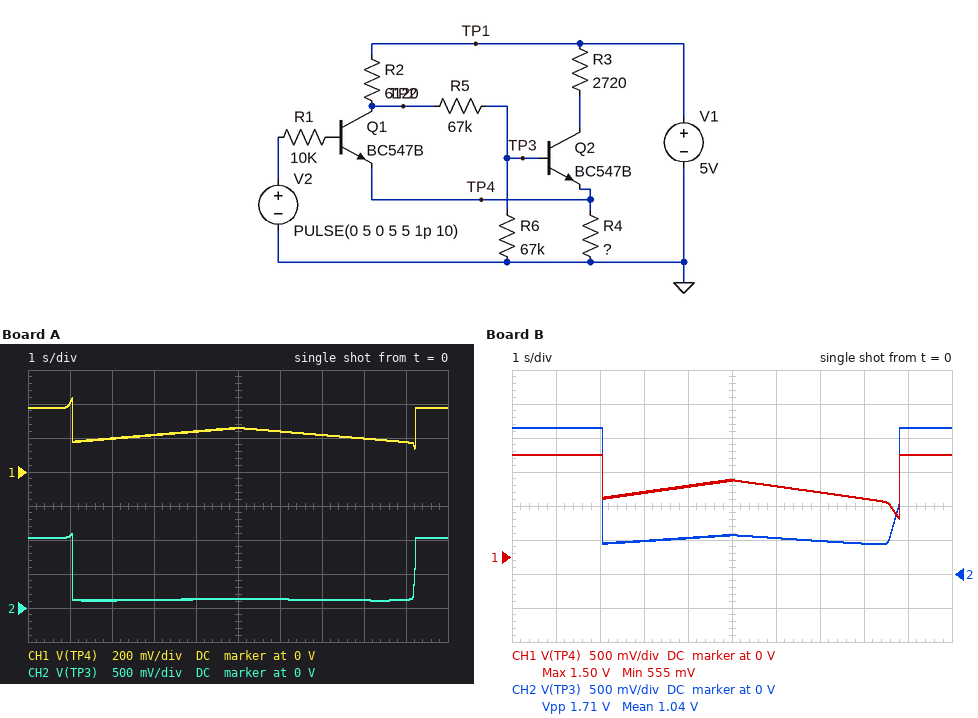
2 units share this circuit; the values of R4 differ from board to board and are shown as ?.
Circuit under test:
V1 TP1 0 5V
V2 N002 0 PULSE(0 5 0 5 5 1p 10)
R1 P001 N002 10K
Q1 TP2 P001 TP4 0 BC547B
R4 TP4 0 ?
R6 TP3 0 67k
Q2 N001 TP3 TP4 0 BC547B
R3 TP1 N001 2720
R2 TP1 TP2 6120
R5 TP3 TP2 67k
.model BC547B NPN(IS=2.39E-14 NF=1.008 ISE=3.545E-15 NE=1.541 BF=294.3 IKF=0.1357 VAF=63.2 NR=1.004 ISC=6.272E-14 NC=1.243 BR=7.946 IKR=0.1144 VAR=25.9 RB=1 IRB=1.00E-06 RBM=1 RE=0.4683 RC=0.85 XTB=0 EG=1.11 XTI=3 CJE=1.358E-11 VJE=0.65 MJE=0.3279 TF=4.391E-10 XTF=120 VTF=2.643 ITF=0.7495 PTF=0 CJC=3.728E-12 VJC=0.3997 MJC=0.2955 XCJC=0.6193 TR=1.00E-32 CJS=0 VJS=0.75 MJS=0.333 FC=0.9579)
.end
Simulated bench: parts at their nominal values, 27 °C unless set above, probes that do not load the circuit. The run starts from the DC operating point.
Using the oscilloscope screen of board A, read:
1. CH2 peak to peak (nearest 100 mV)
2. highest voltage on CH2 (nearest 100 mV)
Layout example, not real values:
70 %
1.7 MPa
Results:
1.0 V
1.1 V
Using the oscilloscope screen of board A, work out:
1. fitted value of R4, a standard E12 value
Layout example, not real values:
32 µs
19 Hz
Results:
220 Ω
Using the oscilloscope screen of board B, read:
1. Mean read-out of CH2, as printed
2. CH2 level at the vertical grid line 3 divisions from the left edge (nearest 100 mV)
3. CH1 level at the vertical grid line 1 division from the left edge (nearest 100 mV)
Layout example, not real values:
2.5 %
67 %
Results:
1.04 V
500 mV
1.5 V
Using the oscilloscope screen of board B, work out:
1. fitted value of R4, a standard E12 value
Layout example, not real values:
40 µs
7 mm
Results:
1.2 kΩ
